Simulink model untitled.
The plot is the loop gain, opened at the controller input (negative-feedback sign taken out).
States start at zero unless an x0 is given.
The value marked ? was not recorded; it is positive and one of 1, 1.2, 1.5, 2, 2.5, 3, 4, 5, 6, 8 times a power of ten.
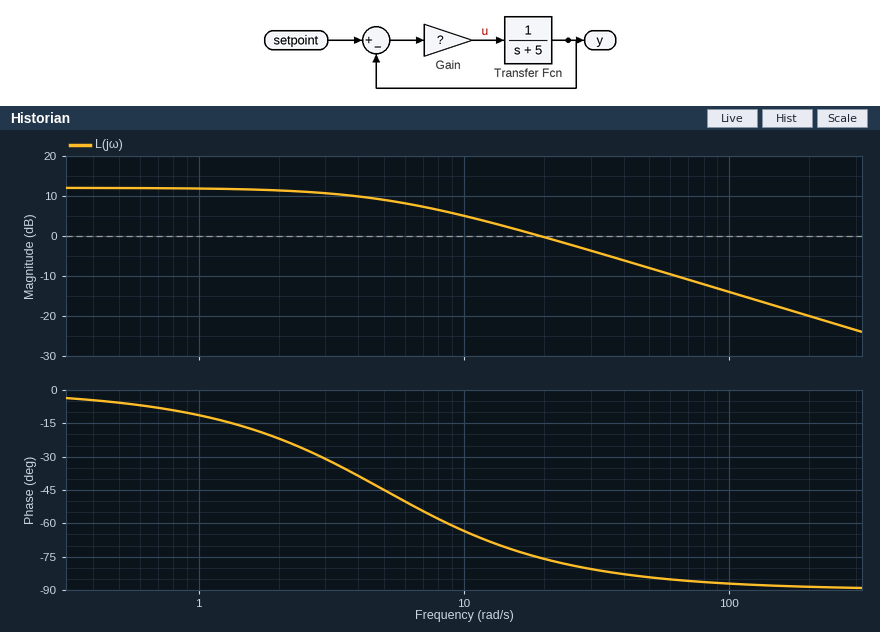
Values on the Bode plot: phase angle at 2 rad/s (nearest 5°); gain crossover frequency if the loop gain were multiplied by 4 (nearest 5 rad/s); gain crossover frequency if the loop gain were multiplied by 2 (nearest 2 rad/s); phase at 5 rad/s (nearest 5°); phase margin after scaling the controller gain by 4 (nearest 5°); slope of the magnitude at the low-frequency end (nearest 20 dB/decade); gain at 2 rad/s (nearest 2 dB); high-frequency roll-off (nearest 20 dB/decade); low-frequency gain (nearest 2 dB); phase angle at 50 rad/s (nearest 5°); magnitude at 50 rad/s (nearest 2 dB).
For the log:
-20°
80 rad/s
40 rad/s
-45°
95°
0 dB/decade
12 dB
-20 dB/decade
12 dB
-85°
-8 dB
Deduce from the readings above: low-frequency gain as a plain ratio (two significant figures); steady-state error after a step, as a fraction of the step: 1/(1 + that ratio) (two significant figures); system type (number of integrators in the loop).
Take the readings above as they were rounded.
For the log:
4.0
0.20
0
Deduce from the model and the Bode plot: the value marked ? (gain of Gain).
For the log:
20
